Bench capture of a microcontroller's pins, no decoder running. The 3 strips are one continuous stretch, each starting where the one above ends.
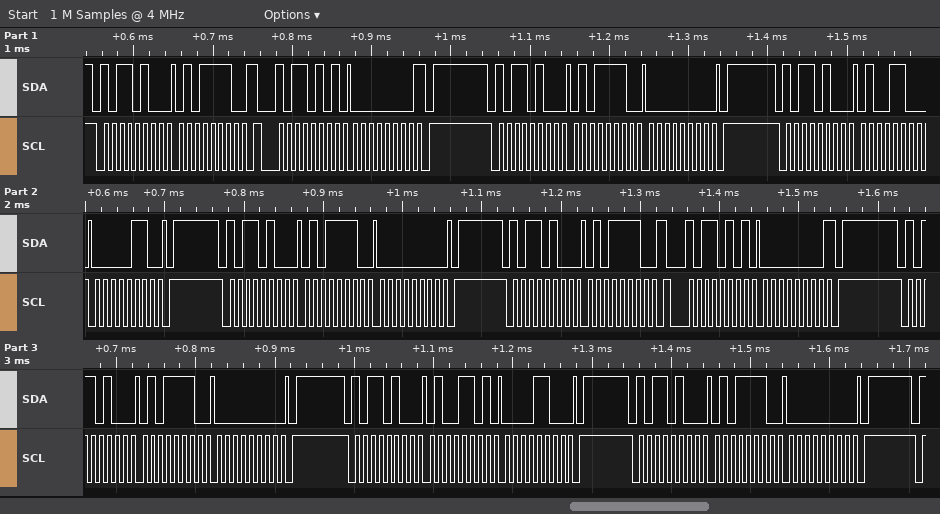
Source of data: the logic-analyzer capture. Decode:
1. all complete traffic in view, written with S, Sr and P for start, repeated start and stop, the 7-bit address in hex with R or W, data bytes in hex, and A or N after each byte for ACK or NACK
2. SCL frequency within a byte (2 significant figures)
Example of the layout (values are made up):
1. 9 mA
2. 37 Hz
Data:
1. S 5AW A 5E A Sr 5AR A 00 N P S 5AW A 5E A 00 A P S 5AW A 4C A 06 A P S 5AW A 5E A 00 A P S 5AW A 5E A Sr 5AR A 00 N P S 5AW A 5E A 00 A P S 5AW A 4D A 0C A P S 5AW A 5E A 00 A P
2. 100 kHz
